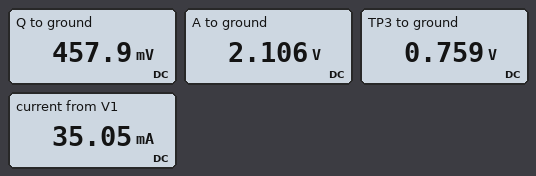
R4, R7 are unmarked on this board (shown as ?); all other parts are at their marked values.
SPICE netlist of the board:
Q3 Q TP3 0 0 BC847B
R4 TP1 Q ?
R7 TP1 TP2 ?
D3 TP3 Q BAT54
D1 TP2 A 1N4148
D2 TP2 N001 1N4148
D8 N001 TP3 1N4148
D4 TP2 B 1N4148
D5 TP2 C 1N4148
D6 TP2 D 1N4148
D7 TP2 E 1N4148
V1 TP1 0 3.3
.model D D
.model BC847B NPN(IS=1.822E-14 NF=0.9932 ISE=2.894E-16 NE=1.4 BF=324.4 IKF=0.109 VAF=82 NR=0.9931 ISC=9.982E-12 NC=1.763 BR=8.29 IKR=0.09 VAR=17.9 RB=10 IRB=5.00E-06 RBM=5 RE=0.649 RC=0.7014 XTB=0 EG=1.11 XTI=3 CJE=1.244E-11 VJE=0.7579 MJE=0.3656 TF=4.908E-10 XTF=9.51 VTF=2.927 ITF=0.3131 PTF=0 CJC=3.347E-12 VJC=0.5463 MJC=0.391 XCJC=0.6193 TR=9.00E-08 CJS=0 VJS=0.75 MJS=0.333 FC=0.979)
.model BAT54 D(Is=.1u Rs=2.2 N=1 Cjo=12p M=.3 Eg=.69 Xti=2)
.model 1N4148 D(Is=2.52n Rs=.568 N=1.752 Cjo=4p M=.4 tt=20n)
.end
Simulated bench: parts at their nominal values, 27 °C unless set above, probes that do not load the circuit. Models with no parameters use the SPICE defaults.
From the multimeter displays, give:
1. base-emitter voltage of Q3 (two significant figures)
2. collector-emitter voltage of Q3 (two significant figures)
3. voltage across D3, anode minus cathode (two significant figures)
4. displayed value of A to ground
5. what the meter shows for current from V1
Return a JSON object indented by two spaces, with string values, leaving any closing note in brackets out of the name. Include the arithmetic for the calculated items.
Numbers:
{
  "base-emitter voltage of Q3": "759 mV = 760 mV",
  "collector-emitter voltage of Q3": "457.9 mV = 460 mV",
  "voltage across D3, anode minus cathode": "759 mV - 457.9 mV = 300 mV",
  "displayed value of A to ground": "2.106 V",
  "what the meter shows for current from V1": "35.05 mA"
}
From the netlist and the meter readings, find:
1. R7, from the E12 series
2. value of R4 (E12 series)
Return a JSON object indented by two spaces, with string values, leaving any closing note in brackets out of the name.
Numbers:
{
  "R7, from the E12 series": "180 Ω",
  "value of R4": "100 Ω"
}
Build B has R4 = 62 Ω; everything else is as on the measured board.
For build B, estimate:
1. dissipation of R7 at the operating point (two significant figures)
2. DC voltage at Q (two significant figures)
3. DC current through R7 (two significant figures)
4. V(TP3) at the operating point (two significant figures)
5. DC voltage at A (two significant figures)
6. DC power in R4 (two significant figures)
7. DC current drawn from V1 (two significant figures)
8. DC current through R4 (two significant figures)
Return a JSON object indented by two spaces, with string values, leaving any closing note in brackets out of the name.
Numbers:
{
  "dissipation of R7 at the operating point": "7.6 mW",
  "DC voltage at Q": "480 mV",
  "DC current through R7": "6.5 mA",
  "V(TP3) at the operating point": "780 mV",
  "DC voltage at A": "2.1 V",
  "DC power in R4": "130 mW",
  "DC current drawn from V1": "52 mA",
  "DC current through R4": "45 mA"
}
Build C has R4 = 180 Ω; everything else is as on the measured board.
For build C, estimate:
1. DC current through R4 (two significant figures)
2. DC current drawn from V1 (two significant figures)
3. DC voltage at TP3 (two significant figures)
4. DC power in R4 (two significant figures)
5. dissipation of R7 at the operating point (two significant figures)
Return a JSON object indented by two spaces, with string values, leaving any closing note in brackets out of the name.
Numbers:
{
  "DC current through R4": "16 mA",
  "DC current drawn from V1": "23 mA",
  "DC voltage at TP3": "740 mV",
  "DC power in R4": "46 mW",
  "dissipation of R7 at the operating point": "8.2 mW"
}
